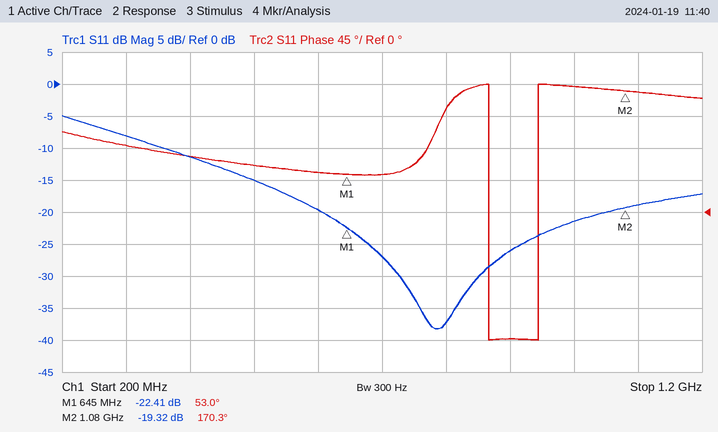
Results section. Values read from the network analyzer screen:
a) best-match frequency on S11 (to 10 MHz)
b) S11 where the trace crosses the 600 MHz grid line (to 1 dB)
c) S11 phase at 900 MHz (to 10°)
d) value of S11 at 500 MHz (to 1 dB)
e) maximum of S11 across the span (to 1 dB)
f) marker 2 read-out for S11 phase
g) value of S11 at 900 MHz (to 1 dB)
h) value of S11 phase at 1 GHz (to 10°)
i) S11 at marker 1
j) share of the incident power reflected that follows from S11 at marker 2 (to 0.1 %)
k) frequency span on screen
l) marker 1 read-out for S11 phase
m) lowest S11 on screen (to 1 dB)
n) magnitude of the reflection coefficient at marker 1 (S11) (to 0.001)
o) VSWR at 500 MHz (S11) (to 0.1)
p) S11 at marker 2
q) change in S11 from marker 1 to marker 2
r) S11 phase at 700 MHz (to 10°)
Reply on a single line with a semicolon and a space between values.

780 MHz; -20 dB; -180°; -15 dB; -5 dB; 170.3°; -26 dB; 180°; -22.41 dB; 1.2 %; 1 GHz; 53.0°; -38 dB; 0.076; 1.4; -19.32 dB; 3.09 dB; 50°
